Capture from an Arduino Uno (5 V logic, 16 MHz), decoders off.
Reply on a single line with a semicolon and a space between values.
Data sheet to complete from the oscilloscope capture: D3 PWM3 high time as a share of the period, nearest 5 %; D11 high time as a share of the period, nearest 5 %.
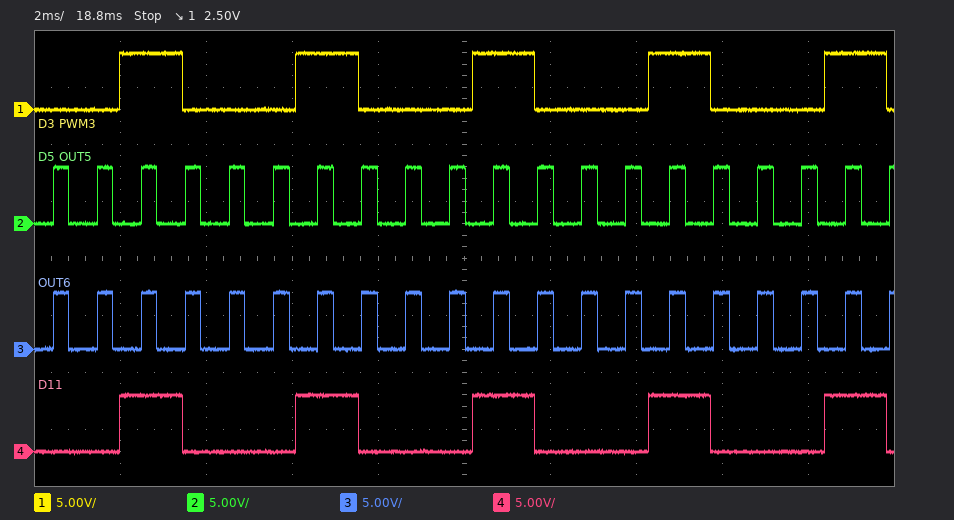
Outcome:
35 %; 35 %
